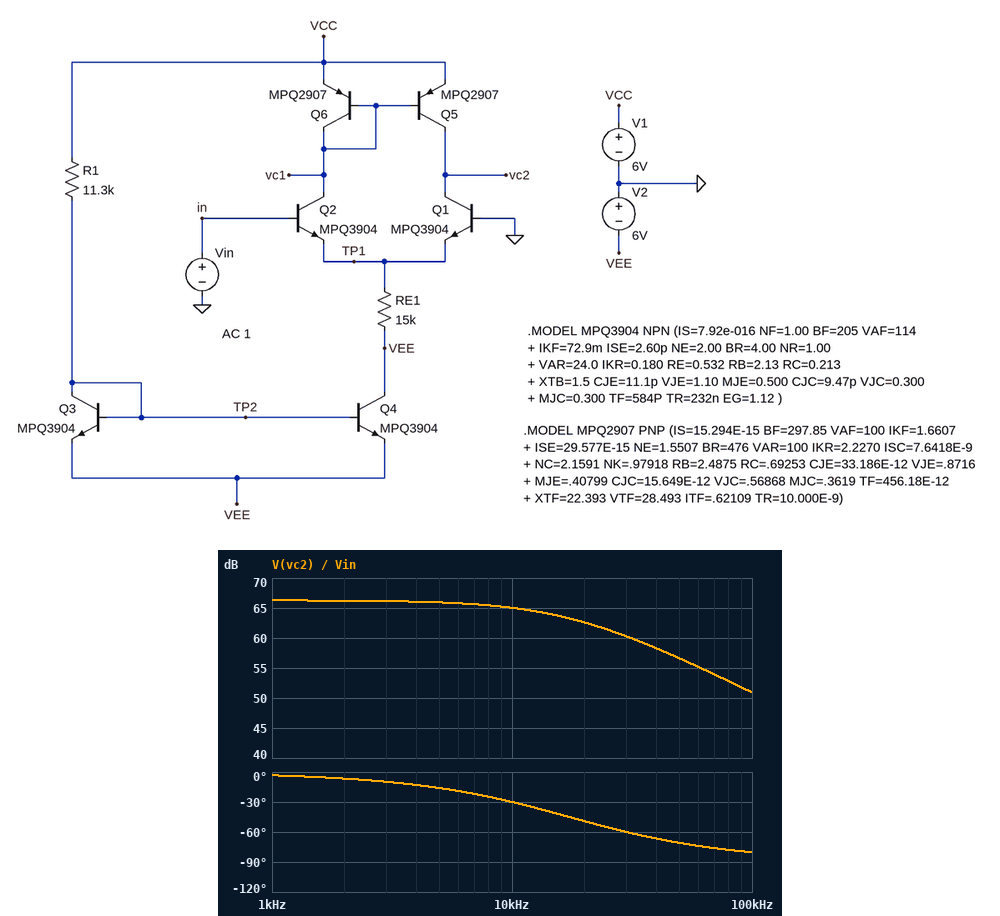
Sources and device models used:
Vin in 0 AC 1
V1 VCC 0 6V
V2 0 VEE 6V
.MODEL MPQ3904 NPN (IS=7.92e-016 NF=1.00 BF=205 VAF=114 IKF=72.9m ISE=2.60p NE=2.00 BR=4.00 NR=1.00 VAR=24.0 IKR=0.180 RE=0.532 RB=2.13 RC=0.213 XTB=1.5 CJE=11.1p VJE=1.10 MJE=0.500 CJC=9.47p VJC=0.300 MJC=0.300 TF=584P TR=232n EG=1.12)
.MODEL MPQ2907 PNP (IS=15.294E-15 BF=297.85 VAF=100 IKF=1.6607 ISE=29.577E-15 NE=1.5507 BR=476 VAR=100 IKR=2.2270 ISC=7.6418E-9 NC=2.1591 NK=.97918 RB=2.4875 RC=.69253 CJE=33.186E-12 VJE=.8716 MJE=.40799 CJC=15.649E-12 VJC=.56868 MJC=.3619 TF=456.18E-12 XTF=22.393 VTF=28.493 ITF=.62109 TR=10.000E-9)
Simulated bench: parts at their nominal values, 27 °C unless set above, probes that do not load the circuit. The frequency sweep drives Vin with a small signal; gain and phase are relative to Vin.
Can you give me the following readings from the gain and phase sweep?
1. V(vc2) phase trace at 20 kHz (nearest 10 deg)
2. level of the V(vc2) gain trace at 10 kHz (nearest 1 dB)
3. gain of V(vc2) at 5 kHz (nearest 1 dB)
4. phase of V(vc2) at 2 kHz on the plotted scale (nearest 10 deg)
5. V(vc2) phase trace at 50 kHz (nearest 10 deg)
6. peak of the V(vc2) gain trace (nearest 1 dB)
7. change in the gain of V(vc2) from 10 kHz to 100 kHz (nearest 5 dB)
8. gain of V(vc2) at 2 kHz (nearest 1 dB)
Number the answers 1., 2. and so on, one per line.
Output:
1. -50 deg
2. 65 dB
3. 66 dB
4. -10 deg
5. -70 deg
6. 66 dB
7. -15 dB
8. 66 dB
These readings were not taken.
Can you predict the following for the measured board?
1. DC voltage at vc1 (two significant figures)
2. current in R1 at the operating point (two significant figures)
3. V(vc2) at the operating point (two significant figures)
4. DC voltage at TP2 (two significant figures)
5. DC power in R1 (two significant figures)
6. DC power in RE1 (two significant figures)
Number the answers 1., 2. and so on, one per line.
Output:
1. 5.4 V
2. 1.0 mA
3. 5.0 V
4. -5.3 V
5. 11 mW
6. 1.9 mW
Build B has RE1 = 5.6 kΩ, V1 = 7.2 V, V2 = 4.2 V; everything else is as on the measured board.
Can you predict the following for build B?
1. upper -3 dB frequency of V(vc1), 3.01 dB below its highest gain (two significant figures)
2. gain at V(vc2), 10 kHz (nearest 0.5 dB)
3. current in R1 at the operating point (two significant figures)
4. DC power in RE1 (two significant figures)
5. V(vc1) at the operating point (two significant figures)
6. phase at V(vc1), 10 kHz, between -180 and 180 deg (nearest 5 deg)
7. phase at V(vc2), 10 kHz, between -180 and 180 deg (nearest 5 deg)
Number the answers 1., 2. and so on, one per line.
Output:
1. 33 kHz
2. 66.0 dB
3. 950 µA
4. 2.2 mW
5. 6.6 V
6. 165 deg
7. -20 deg
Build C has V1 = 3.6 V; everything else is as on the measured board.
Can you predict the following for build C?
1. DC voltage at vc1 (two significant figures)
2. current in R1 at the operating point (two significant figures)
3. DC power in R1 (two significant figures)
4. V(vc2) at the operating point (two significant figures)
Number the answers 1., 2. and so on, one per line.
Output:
1. 3.0 V
2. 790 µA
3. 7.0 mW
4. 2.6 V
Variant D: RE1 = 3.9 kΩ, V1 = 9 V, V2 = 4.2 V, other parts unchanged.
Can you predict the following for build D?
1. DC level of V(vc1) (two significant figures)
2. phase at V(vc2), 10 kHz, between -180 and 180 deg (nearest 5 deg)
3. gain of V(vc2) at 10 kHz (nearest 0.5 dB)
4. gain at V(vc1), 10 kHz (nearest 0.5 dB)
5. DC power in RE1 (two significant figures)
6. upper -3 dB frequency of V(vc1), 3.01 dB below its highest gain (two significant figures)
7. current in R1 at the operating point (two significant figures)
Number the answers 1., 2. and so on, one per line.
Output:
1. 8.4 V
2. -15 deg
3. 66.0 dB
4. -11.5 dB
5. 3.1 mW
6. 47 kHz
7. 1.1 mA
